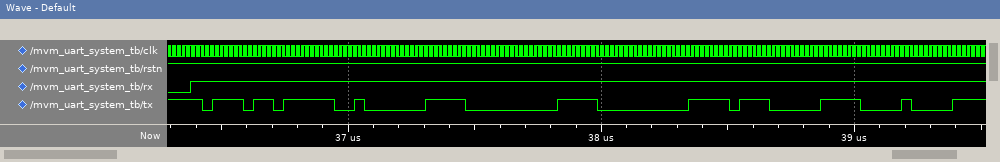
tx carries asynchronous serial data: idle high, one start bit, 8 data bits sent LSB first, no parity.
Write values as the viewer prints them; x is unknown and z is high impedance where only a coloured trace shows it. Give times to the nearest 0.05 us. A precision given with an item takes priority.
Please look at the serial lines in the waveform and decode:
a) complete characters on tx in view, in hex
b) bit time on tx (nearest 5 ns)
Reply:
B7, 02, 00, 00, 07, 08
40 ns
